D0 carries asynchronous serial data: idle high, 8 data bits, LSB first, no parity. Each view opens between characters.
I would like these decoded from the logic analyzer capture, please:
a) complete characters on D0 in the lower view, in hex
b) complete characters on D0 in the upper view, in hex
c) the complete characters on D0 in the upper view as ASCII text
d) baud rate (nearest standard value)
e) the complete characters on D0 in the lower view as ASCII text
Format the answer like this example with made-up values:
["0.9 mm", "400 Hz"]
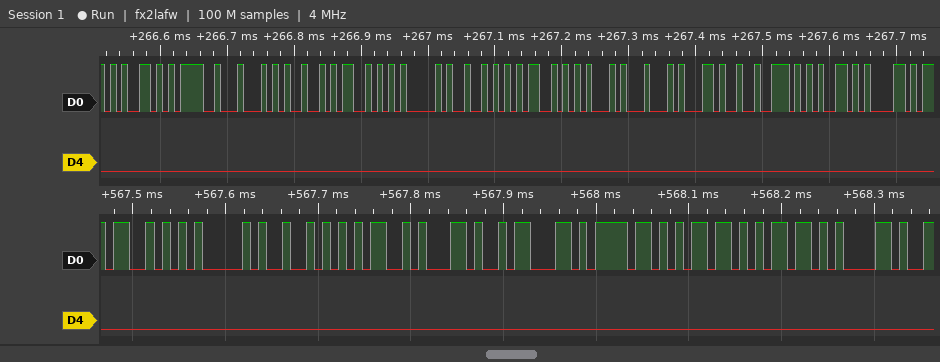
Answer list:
["53, 41, 52, 4D, 2C, 63, 6F, 6D, 6D, 61", "65, 3D, 44, 49, 53, 41, 52, 4D, 45, 44, 2C, 72, 65, 61", "\"e=DISARMED,rea\"", "115200 baud", "\"SARM,comma\""]
